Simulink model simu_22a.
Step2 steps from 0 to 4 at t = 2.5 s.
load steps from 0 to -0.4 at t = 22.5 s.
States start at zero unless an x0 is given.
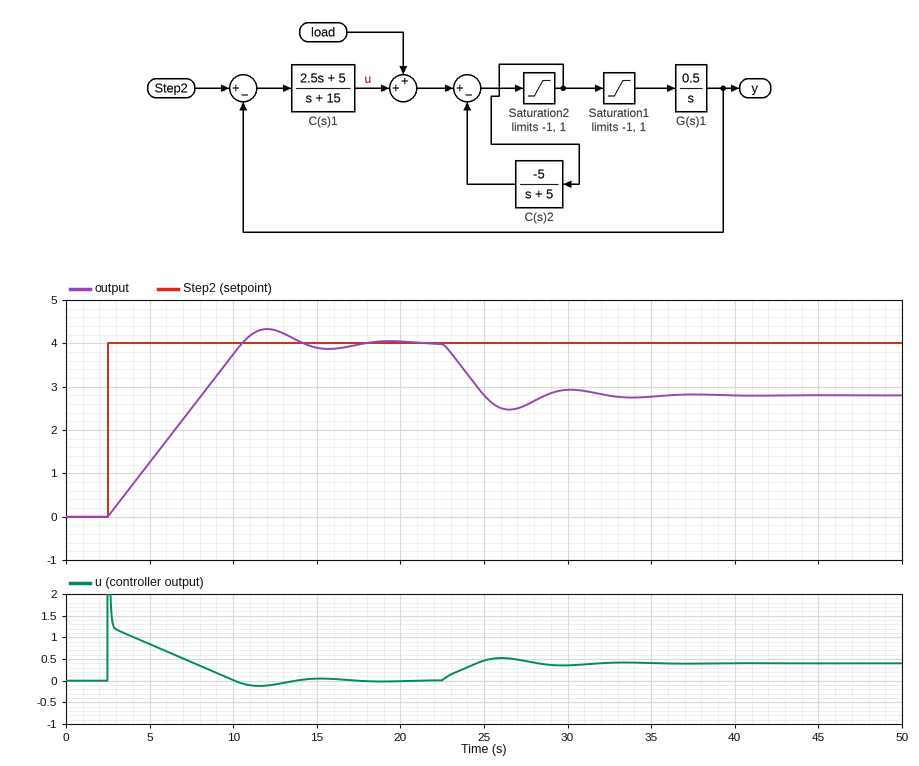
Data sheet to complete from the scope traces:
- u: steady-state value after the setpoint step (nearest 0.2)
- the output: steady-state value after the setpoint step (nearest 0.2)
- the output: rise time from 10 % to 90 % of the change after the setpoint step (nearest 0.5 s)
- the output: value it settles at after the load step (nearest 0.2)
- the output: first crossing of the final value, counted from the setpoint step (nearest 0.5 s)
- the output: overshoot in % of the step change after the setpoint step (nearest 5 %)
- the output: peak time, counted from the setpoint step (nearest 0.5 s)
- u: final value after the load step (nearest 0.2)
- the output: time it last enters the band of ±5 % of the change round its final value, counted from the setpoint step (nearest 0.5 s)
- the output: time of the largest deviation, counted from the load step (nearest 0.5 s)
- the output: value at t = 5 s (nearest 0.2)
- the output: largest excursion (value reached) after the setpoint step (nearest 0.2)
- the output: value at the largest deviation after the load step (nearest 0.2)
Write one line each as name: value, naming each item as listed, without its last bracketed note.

u: steady-state value after the setpoint step: 0.0
the output: steady-state value after the setpoint step: 4.0
the output: rise time from 10 % to 90 % of the change after the setpoint step: 6.5 s
the output: value it settles at after the load step: 2.8
the output: first crossing of the final value, counted from the setpoint step: 8.0 s
the output: overshoot in % of the step change after the setpoint step: 10 %
the output: peak time, counted from the setpoint step: 9.5 s
u: final value after the load step: 0.4
the output: time it last enters the band of ±5 % of the change round its final value, counted from the setpoint step: 10.5 s
the output: time of the largest deviation, counted from the load step: 4.0 s
the output: value at t = 5 s: 1.2
the output: largest excursion (value reached) after the setpoint step: 4.4
the output: value at the largest deviation after the load step: 2.4
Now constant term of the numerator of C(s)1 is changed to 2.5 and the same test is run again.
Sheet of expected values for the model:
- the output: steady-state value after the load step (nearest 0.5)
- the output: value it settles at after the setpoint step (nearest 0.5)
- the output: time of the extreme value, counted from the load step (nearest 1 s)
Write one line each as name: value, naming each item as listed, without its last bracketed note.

the output: steady-state value after the load step: 1.5
the output: value it settles at after the setpoint step: 4.0
the output: time of the extreme value, counted from the load step: 7 s
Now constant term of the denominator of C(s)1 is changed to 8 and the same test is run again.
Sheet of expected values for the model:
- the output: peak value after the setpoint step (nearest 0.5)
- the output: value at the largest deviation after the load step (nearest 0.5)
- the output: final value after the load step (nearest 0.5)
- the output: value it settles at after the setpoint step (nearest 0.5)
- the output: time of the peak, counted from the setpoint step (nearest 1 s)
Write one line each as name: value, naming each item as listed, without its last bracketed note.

the output: peak value after the setpoint step: 4.0
the output: value at the largest deviation after the load step: 3.0
the output: final value after the load step: 3.5
the output: value it settles at after the setpoint step: 4.0
the output: time of the peak, counted from the setpoint step: 9 s
